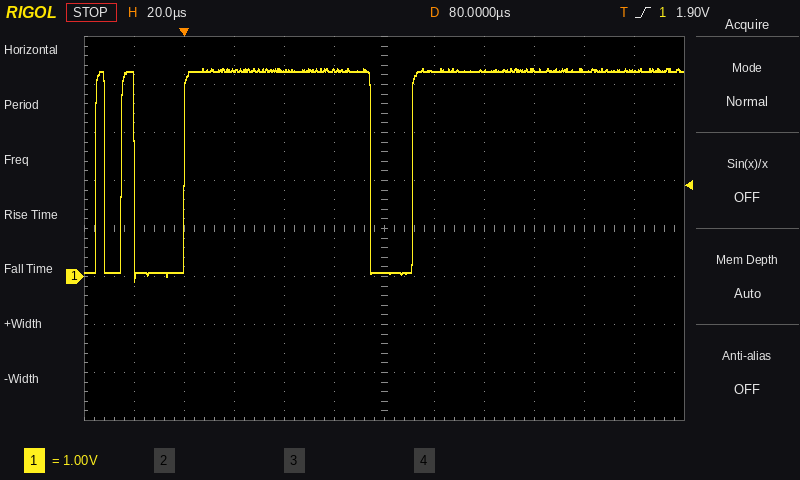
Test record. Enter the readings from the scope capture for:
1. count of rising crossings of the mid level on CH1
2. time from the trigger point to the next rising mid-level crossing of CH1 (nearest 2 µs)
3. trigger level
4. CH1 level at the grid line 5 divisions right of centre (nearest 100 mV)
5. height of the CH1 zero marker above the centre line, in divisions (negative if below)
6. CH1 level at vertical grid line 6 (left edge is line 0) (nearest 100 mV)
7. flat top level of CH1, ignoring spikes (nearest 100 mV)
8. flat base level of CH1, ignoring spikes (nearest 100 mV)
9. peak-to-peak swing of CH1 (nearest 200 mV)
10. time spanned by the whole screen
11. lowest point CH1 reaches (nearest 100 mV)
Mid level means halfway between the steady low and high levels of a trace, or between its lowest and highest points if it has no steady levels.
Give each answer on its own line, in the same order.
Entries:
4
92 µs
1.90 V
4.3 V
-1.0 div
100 mV
4.3 V
100 mV
4.4 V
240 µs
-100 mV
